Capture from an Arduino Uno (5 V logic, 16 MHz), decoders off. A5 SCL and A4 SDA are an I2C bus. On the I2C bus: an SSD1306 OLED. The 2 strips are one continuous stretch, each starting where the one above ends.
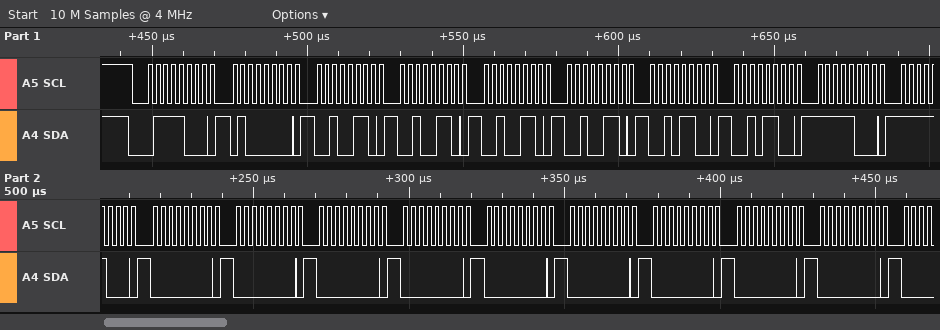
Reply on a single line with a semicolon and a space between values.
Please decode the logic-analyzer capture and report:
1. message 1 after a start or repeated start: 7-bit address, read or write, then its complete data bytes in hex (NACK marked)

0x3C write: 40 26 26 26 26 2C 2C F8 F8 00 00 00 00 00 00 00 00 00
